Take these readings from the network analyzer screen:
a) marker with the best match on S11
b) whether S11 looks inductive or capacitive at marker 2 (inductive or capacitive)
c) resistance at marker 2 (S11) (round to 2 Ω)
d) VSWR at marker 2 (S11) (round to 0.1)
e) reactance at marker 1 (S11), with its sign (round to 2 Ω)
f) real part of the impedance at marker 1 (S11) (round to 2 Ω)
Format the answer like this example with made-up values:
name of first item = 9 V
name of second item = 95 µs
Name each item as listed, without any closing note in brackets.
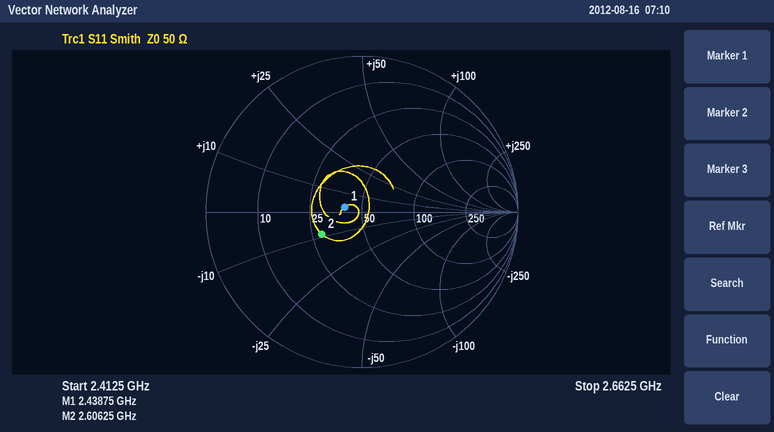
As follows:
marker with the best match on S11 = marker 1
whether S11 looks inductive or capacitive at marker 2 = capacitive
resistance at marker 2 (S11) = 28 Ω
VSWR at marker 2 (S11) = 1.8
reactance at marker 1 (S11), with its sign = +2 Ω
real part of the impedance at marker 1 (S11) = 40 Ω
